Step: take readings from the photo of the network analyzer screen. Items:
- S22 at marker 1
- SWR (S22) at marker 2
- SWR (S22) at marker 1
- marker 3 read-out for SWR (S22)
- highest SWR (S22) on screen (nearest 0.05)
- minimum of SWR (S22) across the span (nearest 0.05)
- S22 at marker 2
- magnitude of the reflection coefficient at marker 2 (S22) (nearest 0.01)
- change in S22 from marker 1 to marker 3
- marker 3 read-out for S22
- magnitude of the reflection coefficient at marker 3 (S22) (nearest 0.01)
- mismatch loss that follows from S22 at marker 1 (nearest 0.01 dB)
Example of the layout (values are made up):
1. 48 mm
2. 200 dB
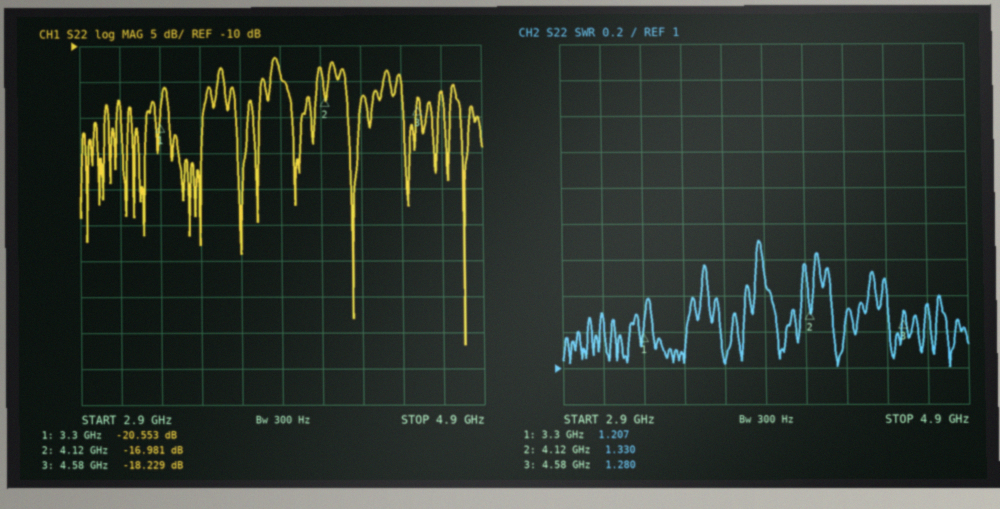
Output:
1. -20.553 dB
2. 1.330
3. 1.207
4. 1.280
5. 1.70
6. 1.00
7. -16.981 dB
8. 0.14
9. 2.324 dB
10. -18.229 dB
11. 0.12
12. 0.04 dB
